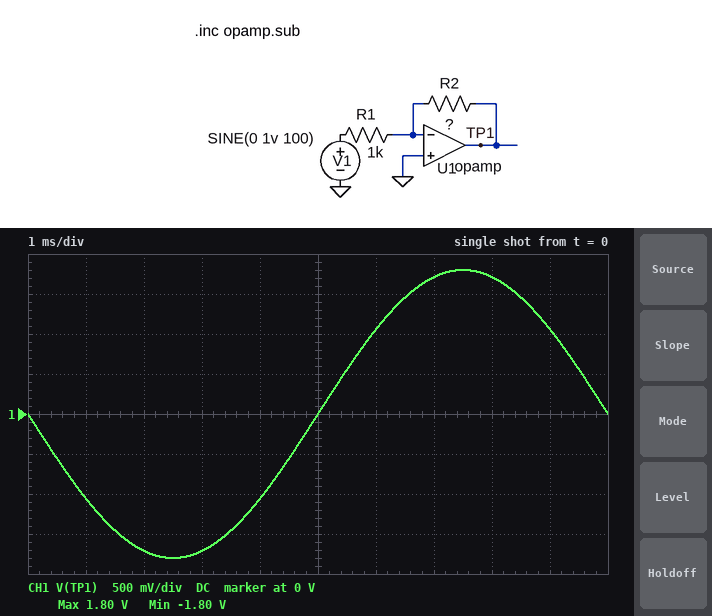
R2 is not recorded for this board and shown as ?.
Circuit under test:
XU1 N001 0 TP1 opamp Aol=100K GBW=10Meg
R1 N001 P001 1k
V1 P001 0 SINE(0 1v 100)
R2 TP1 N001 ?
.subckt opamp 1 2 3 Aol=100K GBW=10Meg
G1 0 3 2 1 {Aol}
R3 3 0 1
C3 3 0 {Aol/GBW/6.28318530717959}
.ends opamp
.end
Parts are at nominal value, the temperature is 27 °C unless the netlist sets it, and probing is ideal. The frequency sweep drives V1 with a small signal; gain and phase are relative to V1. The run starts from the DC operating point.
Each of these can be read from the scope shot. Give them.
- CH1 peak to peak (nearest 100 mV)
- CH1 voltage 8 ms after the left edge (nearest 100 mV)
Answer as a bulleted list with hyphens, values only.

- 3.6 V
- 1.7 V
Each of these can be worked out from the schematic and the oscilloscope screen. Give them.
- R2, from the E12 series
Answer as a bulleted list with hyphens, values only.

- 1.8 kΩ
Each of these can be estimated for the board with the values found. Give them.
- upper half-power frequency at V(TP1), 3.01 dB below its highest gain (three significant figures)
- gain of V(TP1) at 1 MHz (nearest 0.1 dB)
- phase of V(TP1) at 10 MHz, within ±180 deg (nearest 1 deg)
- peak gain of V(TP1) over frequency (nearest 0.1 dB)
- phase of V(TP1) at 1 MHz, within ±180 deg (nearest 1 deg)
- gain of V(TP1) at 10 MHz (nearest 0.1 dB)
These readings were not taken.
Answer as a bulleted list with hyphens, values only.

- 3.57 MHz
- 4.8 dB
- 110 deg
- 5.1 dB
- 164 deg
- -4.4 dB
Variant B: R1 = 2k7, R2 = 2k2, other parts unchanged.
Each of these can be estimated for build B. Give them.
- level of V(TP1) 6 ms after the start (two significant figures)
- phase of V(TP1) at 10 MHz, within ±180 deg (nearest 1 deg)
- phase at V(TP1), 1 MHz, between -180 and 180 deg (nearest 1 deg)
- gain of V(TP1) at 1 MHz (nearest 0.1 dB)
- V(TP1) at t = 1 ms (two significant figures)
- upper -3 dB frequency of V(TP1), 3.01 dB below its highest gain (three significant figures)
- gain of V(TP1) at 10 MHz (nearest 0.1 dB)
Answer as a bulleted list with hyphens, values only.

- 480 mV
- 119 deg
- 170 deg
- -1.9 dB
- -480 mV
- 5.51 MHz
- -8.1 dB
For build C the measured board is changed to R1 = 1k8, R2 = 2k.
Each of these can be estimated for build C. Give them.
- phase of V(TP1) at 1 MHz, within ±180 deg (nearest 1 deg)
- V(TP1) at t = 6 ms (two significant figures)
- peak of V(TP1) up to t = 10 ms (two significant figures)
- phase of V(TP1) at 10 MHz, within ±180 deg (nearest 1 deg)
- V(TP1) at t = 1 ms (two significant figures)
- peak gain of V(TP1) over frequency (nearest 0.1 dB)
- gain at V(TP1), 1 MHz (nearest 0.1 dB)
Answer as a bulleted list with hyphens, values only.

- 168 deg
- 650 mV
- 1.1 V
- 115 deg
- -650 mV
- 0.9 dB
- 0.7 dB
